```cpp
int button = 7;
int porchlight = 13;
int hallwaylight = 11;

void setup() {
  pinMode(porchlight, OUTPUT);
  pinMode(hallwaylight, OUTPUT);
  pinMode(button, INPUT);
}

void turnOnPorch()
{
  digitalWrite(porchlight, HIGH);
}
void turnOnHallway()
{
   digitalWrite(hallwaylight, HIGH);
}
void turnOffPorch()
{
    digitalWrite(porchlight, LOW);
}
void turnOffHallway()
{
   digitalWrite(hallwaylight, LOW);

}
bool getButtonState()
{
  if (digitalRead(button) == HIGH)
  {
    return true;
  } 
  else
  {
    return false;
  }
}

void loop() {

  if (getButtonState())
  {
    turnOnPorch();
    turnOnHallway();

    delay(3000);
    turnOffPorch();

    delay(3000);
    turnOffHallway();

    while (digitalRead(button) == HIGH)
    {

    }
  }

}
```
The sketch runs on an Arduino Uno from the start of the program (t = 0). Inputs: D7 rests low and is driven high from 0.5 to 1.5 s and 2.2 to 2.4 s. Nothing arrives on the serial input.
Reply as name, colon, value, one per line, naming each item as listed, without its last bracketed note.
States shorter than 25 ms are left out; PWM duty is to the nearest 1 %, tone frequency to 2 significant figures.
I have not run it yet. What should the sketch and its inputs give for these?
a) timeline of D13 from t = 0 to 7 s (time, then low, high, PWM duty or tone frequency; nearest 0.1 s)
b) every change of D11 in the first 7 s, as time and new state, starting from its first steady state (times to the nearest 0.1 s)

timeline of D13 from t = 0 to 7 s: 0 s low; 0.5 s high; 3.5 s low
every change of D11 in the first 7 s, as time and new state, starting from its first steady state: 0 s low; 0.5 s high; 6.5 s low
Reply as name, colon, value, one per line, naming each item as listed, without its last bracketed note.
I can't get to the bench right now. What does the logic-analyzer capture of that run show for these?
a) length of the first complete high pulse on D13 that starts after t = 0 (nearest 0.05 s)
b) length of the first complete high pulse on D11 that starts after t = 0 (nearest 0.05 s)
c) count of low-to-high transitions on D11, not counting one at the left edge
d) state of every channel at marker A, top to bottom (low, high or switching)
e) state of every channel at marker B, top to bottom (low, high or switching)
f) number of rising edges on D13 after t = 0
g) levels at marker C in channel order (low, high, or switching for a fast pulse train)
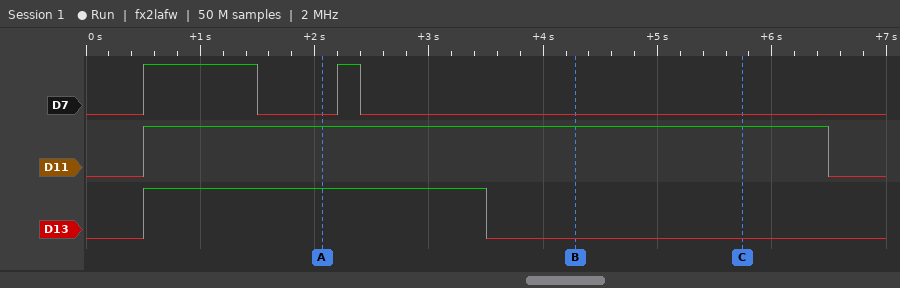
length of the first complete high pulse on D13 that starts after t = 0: 3.00 s
length of the first complete high pulse on D11 that starts after t = 0: 6.00 s
count of low-to-high transitions on D11, not counting one at the left edge: 1
state of every channel at marker A, top to bottom: D7 low, D11 high, D13 high
state of every channel at marker B, top to bottom: D7 low, D11 high, D13 low
number of rising edges on D13 after t = 0: 1
levels at marker C in channel order: D7 low, D11 high, D13 low
